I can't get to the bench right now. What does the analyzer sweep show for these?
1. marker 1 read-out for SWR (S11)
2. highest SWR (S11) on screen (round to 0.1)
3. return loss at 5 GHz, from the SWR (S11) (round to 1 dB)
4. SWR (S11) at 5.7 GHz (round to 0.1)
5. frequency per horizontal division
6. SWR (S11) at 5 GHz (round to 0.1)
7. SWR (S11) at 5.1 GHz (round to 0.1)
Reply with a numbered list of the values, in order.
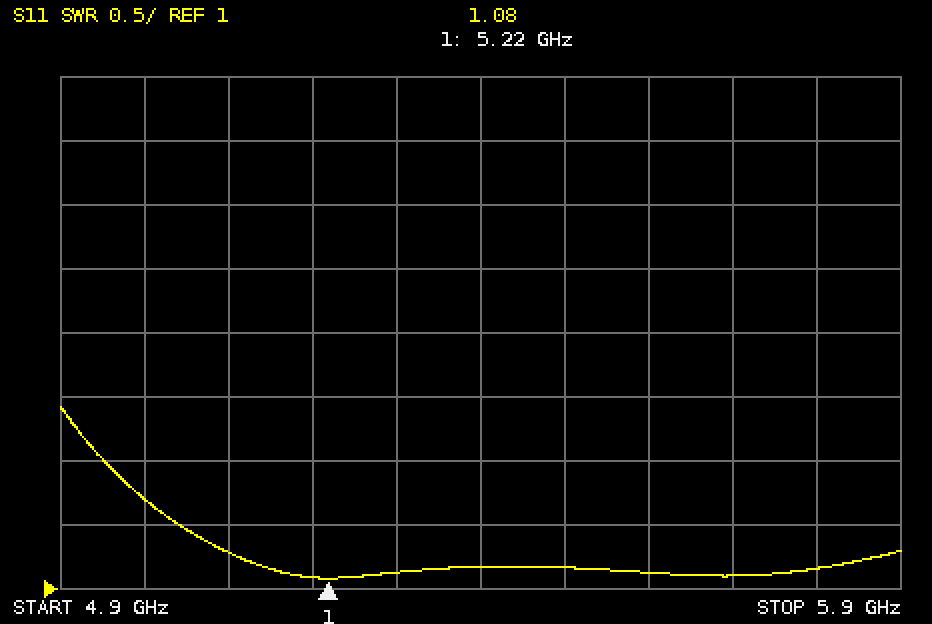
1. 1.08
2. 2.4
3. 12 dB
4. 1.1
5. 100 MHz
6. 1.7
7. 1.3
